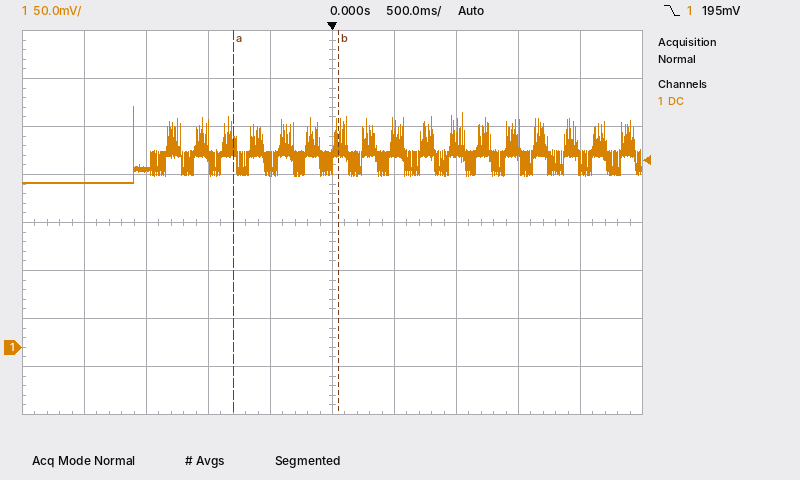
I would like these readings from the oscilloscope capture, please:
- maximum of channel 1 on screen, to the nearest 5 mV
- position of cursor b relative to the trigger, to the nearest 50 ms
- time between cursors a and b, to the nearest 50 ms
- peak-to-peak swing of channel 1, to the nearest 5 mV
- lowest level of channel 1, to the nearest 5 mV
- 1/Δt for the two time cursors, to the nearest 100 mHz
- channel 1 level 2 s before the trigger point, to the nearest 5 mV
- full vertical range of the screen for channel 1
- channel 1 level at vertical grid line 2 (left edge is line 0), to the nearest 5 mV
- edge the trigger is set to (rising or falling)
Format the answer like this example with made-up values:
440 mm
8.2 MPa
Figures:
250 mV
+50 ms
850 ms
80 mV
170 mV
1.2 Hz
170 mV
400 mV
185 mV
falling
